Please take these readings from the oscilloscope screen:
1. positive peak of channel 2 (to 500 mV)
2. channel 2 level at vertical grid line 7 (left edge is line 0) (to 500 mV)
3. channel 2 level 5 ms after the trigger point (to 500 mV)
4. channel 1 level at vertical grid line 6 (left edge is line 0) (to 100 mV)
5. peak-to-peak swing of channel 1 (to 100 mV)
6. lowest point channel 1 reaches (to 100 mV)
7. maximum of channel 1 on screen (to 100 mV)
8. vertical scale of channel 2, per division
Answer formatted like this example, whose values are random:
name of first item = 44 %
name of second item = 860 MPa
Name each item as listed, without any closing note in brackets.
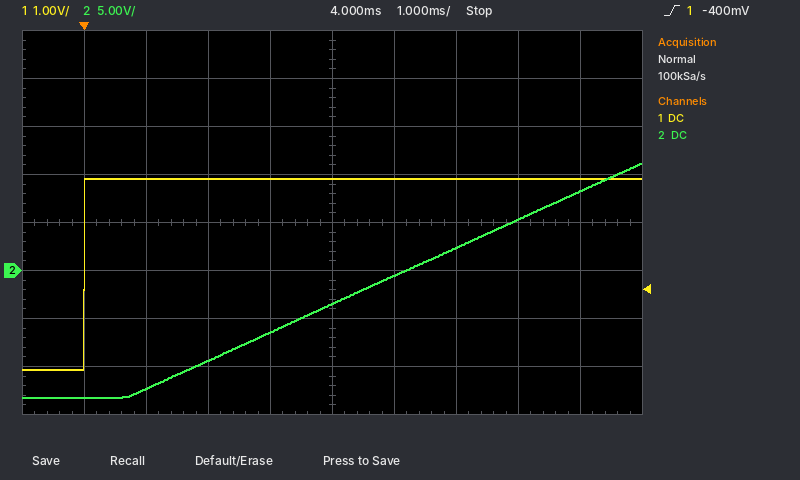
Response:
positive peak of channel 2 = 11.0 V
channel 2 level at vertical grid line 7 (left edge is line 0) = 2.5 V
channel 2 level 5 ms after the trigger point = -500 mV
channel 1 level at vertical grid line 6 (left edge is line 0) = 1.9 V
peak-to-peak swing of channel 1 = 4.0 V
lowest point channel 1 reaches = -2.1 V
maximum of channel 1 on screen = 1.9 V
vertical scale of channel 2, per division = 5 V
